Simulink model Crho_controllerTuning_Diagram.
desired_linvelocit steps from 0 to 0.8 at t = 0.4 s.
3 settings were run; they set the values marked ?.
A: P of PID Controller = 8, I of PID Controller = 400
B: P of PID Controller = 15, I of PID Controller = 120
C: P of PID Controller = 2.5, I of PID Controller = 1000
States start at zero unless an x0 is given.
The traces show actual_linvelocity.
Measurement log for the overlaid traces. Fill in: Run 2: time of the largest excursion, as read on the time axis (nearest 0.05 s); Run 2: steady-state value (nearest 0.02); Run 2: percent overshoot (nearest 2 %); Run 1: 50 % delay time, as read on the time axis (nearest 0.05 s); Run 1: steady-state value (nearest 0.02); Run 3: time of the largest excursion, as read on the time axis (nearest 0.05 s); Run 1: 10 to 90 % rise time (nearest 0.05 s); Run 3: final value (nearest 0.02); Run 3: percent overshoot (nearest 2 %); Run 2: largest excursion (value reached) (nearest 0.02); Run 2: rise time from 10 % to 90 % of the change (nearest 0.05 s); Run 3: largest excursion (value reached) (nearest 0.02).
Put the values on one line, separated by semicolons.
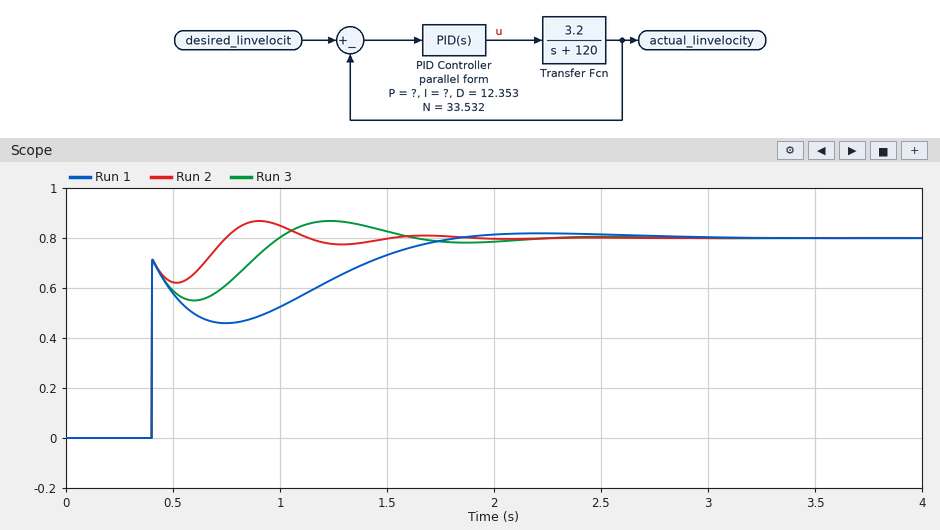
0.90 s; 0.80; 8 %; 0.40 s; 0.80; 1.25 s; 1.05 s; 0.80; 8 %; 0.86; 0.25 s; 0.86
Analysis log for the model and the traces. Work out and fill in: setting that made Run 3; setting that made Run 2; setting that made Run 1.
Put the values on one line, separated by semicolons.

A; C; B
